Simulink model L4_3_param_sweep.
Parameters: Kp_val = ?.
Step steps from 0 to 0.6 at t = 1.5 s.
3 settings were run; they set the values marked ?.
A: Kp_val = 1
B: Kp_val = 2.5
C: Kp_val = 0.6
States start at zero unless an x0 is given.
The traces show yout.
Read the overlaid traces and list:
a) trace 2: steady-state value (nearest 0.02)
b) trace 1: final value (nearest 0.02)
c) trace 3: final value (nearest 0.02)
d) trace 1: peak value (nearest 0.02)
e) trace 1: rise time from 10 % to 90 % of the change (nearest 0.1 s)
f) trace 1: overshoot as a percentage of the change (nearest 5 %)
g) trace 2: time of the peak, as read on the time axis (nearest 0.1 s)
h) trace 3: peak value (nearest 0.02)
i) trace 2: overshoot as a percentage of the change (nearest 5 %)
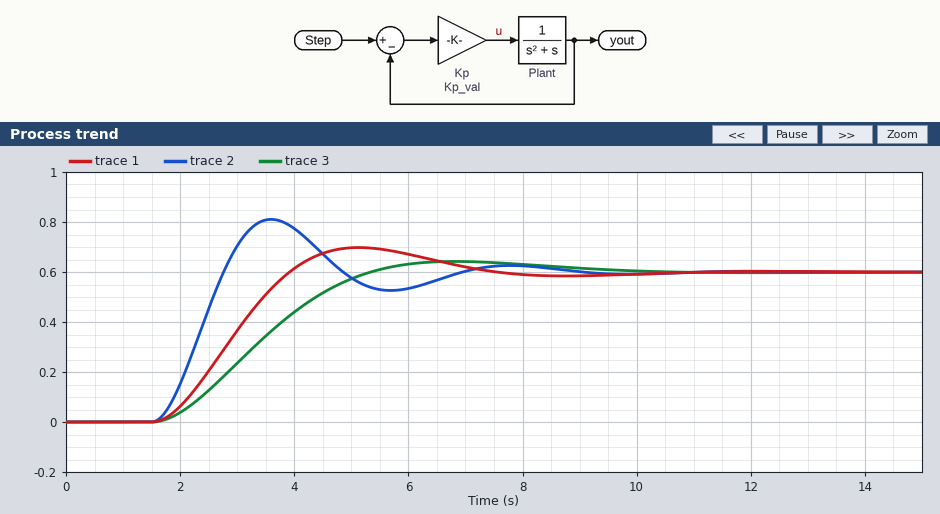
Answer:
0.60
0.60
0.60
0.70
1.6 s
15 %
3.6 s
0.64
35 %
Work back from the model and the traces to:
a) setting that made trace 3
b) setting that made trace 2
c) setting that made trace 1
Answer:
C
B
A
